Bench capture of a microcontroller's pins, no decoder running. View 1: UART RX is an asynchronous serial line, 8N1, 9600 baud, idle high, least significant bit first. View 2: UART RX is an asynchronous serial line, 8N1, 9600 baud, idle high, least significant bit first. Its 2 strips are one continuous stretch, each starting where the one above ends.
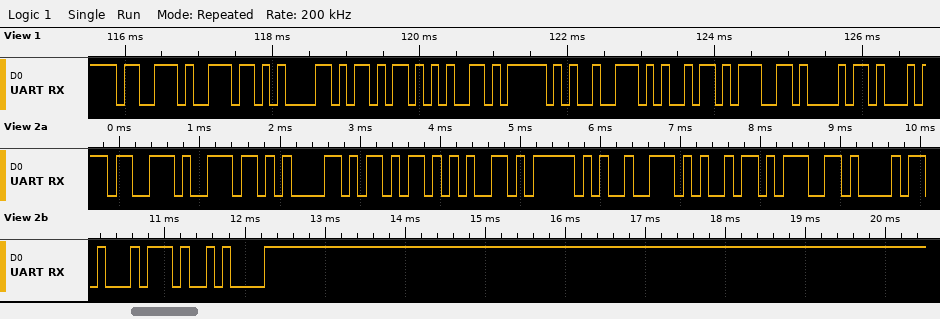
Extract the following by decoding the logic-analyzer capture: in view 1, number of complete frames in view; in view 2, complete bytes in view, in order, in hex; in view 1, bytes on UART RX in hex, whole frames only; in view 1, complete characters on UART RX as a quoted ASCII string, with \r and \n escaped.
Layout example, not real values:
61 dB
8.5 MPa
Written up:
10
73 6E 61 6B 65 5F 72 69 67 68 74 0A
0x73 0x6E 0x61 0x6B 0x65 0x5F 0x72 0x69 0x67 0x68
"snake_righ"
